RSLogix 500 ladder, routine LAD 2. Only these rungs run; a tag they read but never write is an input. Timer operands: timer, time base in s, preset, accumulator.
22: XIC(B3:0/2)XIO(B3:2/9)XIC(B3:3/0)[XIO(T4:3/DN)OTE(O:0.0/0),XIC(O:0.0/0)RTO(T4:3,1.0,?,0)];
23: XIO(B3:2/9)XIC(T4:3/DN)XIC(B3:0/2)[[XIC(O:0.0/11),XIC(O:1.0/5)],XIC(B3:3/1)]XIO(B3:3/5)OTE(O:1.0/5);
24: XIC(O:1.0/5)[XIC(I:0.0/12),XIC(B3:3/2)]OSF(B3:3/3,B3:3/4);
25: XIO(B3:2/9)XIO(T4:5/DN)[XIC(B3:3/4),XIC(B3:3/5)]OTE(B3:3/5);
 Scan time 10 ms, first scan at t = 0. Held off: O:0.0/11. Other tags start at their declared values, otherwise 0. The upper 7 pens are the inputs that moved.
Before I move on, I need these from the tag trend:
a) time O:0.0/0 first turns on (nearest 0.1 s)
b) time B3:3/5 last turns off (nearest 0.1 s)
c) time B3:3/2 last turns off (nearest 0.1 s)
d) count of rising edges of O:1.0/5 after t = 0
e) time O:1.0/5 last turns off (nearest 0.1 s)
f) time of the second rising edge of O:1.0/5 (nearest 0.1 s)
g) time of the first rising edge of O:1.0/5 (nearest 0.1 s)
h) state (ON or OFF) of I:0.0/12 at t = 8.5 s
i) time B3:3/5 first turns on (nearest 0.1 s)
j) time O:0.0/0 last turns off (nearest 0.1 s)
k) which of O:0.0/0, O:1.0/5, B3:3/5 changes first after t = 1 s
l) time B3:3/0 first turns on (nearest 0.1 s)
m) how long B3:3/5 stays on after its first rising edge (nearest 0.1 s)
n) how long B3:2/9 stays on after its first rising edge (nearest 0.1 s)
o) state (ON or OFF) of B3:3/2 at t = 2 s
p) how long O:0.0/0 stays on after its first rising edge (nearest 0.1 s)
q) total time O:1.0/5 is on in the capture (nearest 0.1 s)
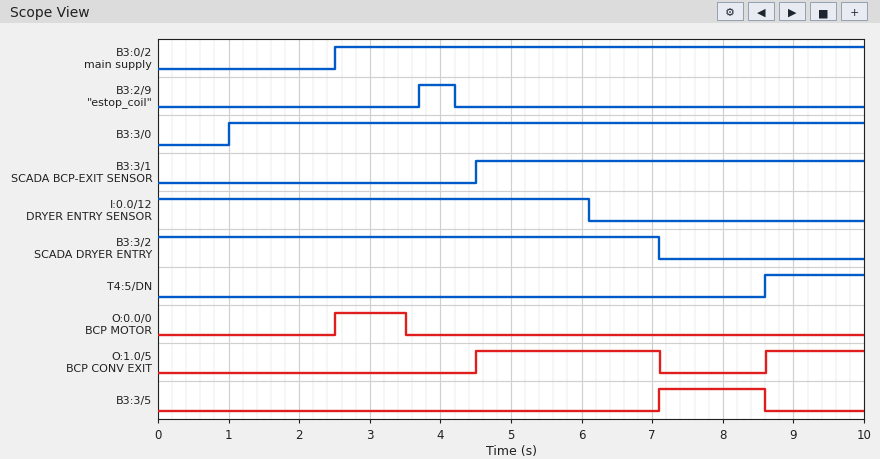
2.5 s
8.6 s
7.1 s
2
7.1 s
8.6 s
4.5 s
OFF
7.1 s
3.5 s
O:0.0/0
1.0 s
1.5 s
0.5 s
ON
1.0 s
4.0 s
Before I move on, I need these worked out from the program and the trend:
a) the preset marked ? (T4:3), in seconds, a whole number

1 s
